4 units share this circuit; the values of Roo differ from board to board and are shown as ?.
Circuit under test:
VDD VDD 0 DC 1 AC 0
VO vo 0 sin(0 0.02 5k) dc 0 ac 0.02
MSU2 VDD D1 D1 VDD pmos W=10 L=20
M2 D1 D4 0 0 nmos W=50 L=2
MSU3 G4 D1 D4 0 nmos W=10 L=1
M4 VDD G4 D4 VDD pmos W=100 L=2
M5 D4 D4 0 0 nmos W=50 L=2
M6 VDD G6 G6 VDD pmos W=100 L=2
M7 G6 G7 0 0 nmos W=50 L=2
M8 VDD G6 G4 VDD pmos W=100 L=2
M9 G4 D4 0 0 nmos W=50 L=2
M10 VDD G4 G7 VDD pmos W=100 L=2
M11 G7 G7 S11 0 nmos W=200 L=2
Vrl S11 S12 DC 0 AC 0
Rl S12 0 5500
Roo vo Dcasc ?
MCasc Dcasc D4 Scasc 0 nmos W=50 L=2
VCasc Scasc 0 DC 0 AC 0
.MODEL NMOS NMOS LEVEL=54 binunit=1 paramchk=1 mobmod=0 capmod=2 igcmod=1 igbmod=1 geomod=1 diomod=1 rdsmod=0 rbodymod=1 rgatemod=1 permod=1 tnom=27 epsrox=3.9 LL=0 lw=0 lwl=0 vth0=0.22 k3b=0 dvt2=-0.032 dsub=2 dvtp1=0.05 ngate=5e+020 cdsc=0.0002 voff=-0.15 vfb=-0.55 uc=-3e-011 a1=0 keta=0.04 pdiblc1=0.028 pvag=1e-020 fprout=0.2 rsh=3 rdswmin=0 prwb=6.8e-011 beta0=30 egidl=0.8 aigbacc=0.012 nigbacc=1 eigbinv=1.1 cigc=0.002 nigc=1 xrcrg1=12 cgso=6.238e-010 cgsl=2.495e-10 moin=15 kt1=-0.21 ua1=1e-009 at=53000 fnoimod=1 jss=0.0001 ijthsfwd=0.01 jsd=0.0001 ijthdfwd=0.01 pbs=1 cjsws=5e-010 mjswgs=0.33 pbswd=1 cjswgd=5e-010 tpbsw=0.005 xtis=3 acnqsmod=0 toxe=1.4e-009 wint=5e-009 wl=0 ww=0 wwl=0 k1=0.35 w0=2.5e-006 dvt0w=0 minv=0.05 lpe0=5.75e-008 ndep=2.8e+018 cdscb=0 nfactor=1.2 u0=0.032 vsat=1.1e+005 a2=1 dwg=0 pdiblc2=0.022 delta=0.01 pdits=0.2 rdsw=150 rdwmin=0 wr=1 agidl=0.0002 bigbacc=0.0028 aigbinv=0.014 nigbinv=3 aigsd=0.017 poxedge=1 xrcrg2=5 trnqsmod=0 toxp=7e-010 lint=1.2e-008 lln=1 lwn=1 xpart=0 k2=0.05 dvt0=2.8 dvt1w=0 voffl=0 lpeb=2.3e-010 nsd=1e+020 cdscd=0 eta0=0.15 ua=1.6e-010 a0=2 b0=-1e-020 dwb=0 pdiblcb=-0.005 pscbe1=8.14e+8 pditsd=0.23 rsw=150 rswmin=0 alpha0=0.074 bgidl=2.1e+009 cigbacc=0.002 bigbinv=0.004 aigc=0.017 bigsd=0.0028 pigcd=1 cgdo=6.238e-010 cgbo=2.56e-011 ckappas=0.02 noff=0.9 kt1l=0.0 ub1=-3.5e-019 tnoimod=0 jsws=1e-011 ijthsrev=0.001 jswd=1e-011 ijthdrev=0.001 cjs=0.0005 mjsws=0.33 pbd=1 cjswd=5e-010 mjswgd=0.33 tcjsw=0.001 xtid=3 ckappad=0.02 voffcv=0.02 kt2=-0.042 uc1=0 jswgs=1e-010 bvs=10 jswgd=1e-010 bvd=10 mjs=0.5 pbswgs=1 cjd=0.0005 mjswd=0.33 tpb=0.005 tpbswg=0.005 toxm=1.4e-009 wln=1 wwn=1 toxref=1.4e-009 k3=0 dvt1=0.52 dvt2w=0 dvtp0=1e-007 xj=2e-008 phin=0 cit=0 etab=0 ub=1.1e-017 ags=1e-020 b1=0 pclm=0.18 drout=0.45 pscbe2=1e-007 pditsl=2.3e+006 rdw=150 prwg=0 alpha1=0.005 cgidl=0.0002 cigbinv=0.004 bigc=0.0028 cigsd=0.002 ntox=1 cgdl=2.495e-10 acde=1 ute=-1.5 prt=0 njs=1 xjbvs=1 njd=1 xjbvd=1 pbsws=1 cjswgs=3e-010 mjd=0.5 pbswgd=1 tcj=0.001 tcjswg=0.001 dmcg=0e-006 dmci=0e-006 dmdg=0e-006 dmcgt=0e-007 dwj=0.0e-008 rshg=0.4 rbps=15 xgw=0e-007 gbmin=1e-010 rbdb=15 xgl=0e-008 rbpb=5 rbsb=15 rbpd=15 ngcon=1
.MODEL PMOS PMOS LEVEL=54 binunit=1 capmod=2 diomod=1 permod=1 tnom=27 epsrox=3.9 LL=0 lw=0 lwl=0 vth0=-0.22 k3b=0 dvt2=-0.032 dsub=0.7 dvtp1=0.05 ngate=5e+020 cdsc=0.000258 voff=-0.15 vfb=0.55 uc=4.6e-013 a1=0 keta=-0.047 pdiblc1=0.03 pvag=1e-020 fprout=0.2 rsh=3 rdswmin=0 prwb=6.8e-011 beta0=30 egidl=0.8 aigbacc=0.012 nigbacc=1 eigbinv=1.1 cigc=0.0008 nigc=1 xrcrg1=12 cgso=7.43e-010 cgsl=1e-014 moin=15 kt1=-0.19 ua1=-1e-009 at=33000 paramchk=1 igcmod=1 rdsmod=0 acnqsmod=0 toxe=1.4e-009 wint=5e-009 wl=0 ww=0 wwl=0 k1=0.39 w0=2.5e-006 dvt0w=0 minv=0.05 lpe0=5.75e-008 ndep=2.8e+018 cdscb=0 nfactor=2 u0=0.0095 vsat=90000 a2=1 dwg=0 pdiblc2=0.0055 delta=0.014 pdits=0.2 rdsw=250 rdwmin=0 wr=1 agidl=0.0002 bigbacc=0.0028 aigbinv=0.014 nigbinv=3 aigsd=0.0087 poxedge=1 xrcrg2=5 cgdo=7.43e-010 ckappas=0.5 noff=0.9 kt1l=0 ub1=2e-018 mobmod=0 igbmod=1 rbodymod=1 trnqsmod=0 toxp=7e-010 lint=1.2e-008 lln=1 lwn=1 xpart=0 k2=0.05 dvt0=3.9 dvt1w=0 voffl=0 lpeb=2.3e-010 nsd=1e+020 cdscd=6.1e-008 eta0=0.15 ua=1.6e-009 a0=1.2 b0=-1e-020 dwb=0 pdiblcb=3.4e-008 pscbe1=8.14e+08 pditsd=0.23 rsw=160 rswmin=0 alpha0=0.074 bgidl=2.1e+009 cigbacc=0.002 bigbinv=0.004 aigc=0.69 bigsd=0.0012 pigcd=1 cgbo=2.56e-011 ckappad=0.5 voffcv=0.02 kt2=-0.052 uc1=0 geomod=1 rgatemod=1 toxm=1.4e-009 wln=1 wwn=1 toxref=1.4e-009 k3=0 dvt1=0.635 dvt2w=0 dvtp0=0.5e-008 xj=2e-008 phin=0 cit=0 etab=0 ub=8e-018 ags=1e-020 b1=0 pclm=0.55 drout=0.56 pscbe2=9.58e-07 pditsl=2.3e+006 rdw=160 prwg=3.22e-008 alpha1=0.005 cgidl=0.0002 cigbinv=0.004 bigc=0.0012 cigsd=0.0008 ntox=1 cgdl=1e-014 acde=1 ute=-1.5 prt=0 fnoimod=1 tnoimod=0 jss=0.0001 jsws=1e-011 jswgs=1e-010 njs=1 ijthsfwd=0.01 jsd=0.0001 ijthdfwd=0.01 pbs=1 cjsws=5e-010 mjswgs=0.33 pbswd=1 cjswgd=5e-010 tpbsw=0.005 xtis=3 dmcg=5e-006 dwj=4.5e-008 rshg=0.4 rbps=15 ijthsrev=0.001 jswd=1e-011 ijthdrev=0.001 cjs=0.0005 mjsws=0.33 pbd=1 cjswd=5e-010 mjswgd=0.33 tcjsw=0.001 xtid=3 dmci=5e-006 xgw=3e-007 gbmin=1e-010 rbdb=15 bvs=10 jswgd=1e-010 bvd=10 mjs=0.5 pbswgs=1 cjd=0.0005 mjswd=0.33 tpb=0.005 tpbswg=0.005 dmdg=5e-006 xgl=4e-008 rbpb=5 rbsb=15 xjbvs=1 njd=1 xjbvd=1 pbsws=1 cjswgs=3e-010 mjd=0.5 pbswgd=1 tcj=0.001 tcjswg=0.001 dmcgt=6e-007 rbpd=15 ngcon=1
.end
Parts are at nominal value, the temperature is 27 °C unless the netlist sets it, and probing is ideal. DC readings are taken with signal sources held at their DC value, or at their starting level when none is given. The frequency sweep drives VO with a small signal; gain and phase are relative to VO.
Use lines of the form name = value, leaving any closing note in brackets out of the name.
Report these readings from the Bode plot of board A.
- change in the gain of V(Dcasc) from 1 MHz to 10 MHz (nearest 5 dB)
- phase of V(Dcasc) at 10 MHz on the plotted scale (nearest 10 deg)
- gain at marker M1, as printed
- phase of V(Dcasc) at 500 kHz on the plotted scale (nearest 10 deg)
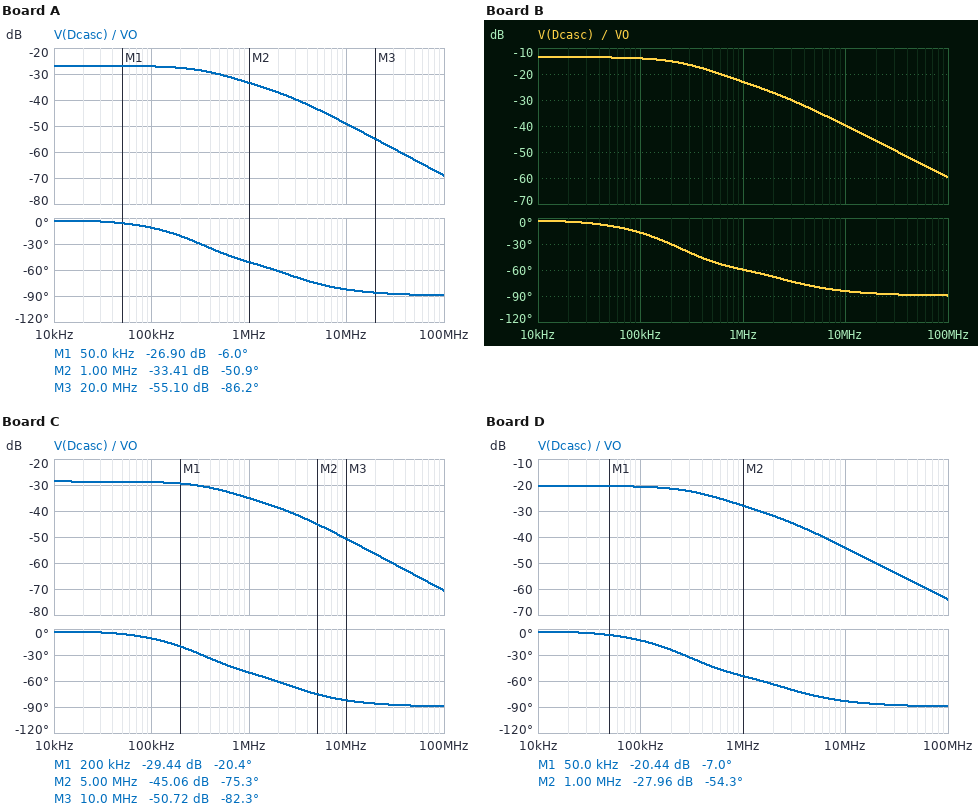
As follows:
change in the gain of V(Dcasc) from 1 MHz to 10 MHz = -15 dB
phase of V(Dcasc) at 10 MHz on the plotted scale = -80 deg
gain at marker M1, as printed = -26.90 dB
phase of V(Dcasc) at 500 kHz on the plotted scale = -40 deg
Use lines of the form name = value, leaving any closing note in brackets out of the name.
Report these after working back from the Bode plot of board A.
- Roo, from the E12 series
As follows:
Roo, from the E12 series = 150 Ω
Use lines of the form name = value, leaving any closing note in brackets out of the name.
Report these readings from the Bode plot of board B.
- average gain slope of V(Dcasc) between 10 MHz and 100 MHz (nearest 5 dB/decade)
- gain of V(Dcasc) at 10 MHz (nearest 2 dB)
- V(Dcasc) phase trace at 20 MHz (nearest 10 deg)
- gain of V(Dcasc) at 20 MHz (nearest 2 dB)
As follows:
average gain slope of V(Dcasc) between 10 MHz and 100 MHz = -20 dB/decade
gain of V(Dcasc) at 10 MHz = -40 dB
V(Dcasc) phase trace at 20 MHz = -90 deg
gain of V(Dcasc) at 20 MHz = -46 dB
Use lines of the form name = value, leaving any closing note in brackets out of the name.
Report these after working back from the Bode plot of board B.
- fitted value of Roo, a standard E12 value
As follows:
fitted value of Roo, a standard E12 value = 47 Ω
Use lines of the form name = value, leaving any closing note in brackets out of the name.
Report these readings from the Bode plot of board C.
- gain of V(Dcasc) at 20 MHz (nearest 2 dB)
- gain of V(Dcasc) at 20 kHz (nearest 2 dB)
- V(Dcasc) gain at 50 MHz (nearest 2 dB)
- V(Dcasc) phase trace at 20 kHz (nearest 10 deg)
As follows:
gain of V(Dcasc) at 20 MHz = -56 dB
gain of V(Dcasc) at 20 kHz = -28 dB
V(Dcasc) gain at 50 MHz = -64 dB
V(Dcasc) phase trace at 20 kHz = 0 deg
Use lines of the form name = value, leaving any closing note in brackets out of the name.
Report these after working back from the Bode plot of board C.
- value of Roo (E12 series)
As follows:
value of Roo = 180 Ω
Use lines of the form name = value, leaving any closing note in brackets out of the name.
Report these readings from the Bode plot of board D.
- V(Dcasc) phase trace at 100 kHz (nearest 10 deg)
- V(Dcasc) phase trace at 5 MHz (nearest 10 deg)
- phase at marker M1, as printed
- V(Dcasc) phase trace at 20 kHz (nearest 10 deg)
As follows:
V(Dcasc) phase trace at 100 kHz = -10 deg
V(Dcasc) phase trace at 5 MHz = -80 deg
phase at marker M1, as printed = -7.0 deg
V(Dcasc) phase trace at 20 kHz = 0 deg
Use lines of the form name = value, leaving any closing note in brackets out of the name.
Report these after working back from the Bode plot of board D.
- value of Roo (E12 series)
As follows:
value of Roo = 82 Ω
